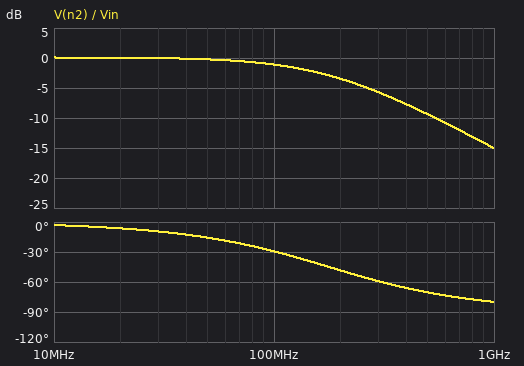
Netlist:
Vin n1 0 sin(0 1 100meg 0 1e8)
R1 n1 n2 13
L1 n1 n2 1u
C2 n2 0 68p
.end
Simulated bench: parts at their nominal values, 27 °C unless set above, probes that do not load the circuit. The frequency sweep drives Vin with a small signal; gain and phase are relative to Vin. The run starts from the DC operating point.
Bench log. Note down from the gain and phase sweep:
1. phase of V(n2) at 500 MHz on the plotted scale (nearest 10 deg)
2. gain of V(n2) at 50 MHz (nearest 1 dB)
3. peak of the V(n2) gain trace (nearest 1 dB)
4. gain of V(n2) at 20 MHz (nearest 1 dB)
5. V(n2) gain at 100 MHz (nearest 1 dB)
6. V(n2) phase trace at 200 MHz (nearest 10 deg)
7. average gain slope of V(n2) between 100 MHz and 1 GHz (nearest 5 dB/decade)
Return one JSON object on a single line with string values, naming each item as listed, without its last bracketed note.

{"phase of V(n2) at 500 MHz on the plotted scale": "-70 deg", "gain of V(n2) at 50 MHz": "0 dB", "peak of the V(n2) gain trace": "0 dB", "gain of V(n2) at 20 MHz": "0 dB", "V(n2) gain at 100 MHz": "-1 dB", "V(n2) phase trace at 200 MHz": "-50 deg", "average gain slope of V(n2) between 100 MHz and 1 GHz": "-15 dB/decade"}
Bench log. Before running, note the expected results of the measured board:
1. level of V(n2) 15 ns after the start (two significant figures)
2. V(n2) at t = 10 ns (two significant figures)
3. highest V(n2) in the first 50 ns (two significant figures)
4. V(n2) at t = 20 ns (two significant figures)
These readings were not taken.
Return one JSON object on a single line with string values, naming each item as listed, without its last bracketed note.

{"level of V(n2) 15 ns after the start": "110 mV", "V(n2) at t = 10 ns": "-180 mV", "highest V(n2) in the first 50 ns": "700 mV", "V(n2) at t = 20 ns": "-67 mV"}
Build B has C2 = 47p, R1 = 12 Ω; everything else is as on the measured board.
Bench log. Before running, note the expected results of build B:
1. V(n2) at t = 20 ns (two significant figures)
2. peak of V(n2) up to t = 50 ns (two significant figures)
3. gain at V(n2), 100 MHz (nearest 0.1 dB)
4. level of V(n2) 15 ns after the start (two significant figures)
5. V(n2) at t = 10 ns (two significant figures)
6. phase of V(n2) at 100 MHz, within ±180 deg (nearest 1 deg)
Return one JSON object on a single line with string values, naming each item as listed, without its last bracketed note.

{"V(n2) at t = 20 ns": "-48 mV", "peak of V(n2) up to t = 50 ns": "750 mV", "gain at V(n2), 100 MHz": "-0.5 dB", "level of V(n2) 15 ns after the start": "79 mV", "V(n2) at t = 10 ns": "-130 mV", "phase of V(n2) at 100 MHz, within ±180 deg": "-20 deg"}
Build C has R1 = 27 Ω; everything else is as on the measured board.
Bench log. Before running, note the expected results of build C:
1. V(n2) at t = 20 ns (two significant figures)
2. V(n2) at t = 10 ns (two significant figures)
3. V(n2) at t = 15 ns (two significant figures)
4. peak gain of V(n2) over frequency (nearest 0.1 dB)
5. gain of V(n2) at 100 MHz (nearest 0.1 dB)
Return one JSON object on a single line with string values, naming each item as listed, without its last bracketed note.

{"V(n2) at t = 20 ns": "-83 mV", "V(n2) at t = 10 ns": "-220 mV", "V(n2) at t = 15 ns": "130 mV", "peak gain of V(n2) over frequency": "0.3 dB", "gain of V(n2) at 100 MHz": "-3.5 dB"}
